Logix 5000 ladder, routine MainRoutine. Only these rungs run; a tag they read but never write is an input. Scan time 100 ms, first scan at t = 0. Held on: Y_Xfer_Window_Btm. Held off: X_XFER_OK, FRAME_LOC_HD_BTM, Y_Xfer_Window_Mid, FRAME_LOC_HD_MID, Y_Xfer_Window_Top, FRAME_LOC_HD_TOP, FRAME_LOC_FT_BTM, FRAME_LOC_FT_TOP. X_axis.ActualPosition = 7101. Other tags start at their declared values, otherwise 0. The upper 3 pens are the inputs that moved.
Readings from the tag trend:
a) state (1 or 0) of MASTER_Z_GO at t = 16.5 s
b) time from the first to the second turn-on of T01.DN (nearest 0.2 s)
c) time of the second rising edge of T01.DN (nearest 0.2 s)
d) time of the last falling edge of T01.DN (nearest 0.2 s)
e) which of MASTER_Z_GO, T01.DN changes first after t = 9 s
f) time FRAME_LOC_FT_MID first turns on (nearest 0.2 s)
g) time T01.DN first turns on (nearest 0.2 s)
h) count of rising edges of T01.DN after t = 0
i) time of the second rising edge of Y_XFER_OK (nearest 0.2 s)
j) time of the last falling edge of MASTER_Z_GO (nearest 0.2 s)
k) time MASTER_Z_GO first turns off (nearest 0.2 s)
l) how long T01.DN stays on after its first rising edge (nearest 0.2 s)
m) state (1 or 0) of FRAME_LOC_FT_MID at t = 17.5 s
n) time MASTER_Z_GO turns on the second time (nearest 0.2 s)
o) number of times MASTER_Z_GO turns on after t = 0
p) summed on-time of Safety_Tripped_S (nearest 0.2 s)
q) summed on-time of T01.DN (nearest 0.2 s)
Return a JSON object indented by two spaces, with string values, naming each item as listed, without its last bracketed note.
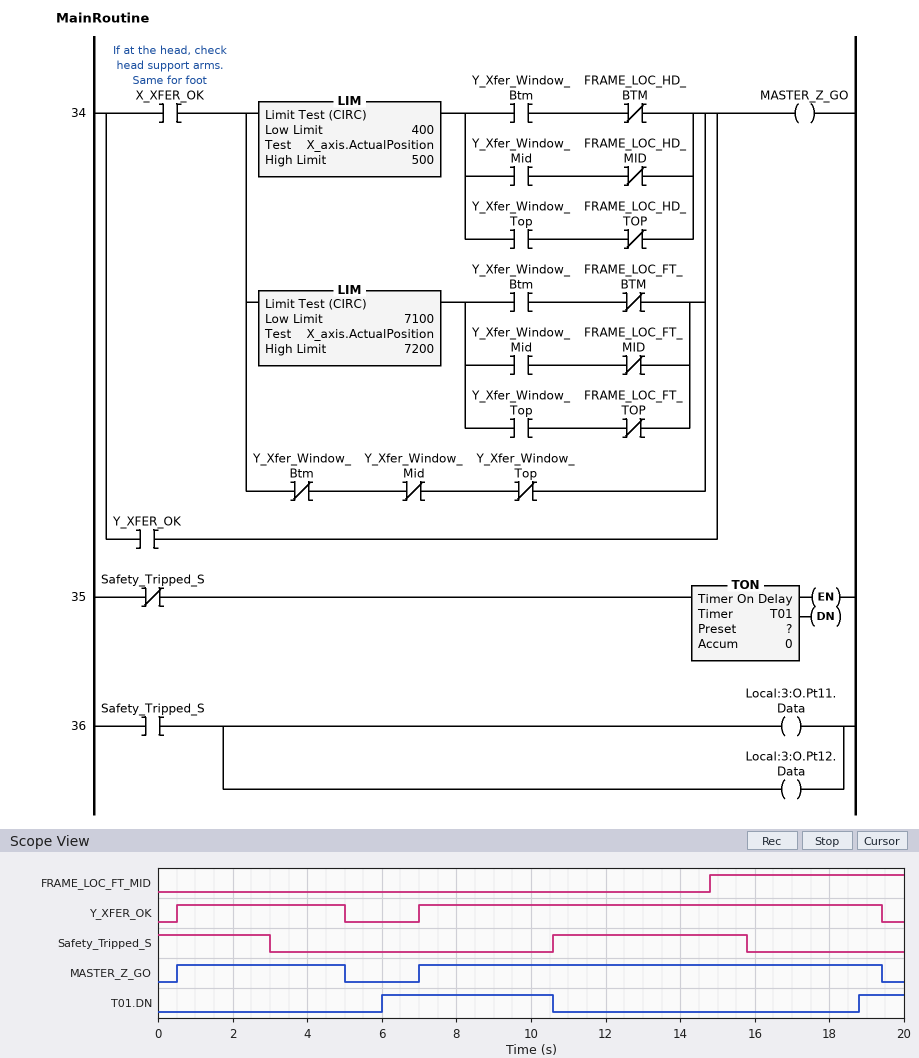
{
  "state (1 or 0) of MASTER_Z_GO at t = 16.5 s": "1",
  "time from the first to the second turn-on of T01.DN": "12.8 s",
  "time of the second rising edge of T01.DN": "18.8 s",
  "time of the last falling edge of T01.DN": "10.6 s",
  "which of MASTER_Z_GO, T01.DN changes first after t = 9 s": "T01.DN",
  "time FRAME_LOC_FT_MID first turns on": "14.8 s",
  "time T01.DN first turns on": "6.0 s",
  "count of rising edges of T01.DN after t = 0": "2",
  "time of the second rising edge of Y_XFER_OK": "7.0 s",
  "time of the last falling edge of MASTER_Z_GO": "19.4 s",
  "time MASTER_Z_GO first turns off": "5.0 s",
  "how long T01.DN stays on after its first rising edge": "4.6 s",
  "state (1 or 0) of FRAME_LOC_FT_MID at t = 17.5 s": "1",
  "time MASTER_Z_GO turns on the second time": "7.0 s",
  "number of times MASTER_Z_GO turns on after t = 0": "2",
  "summed on-time of Safety_Tripped_S": "8.2 s",
  "summed on-time of T01.DN": "5.8 s"
}
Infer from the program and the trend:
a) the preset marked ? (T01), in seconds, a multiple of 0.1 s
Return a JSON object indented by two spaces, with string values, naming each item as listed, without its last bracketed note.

{
  "the preset marked ? (T01), in seconds, a multiple of 0.1 s": "3.0 s"
}
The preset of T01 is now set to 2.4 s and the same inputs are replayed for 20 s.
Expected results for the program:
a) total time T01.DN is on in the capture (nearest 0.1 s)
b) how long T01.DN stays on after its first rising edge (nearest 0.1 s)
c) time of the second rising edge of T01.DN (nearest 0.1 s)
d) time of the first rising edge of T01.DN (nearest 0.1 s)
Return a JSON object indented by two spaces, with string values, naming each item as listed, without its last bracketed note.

{
  "total time T01.DN is on in the capture": "7.0 s",
  "how long T01.DN stays on after its first rising edge": "5.2 s",
  "time of the second rising edge of T01.DN": "18.2 s",
  "time of the first rising edge of T01.DN": "5.4 s"
}
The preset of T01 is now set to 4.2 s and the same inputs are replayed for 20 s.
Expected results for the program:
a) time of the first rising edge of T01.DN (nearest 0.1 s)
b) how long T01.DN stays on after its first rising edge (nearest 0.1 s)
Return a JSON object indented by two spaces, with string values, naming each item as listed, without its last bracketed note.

{
  "time of the first rising edge of T01.DN": "7.2 s",
  "how long T01.DN stays on after its first rising edge": "3.4 s"
}
